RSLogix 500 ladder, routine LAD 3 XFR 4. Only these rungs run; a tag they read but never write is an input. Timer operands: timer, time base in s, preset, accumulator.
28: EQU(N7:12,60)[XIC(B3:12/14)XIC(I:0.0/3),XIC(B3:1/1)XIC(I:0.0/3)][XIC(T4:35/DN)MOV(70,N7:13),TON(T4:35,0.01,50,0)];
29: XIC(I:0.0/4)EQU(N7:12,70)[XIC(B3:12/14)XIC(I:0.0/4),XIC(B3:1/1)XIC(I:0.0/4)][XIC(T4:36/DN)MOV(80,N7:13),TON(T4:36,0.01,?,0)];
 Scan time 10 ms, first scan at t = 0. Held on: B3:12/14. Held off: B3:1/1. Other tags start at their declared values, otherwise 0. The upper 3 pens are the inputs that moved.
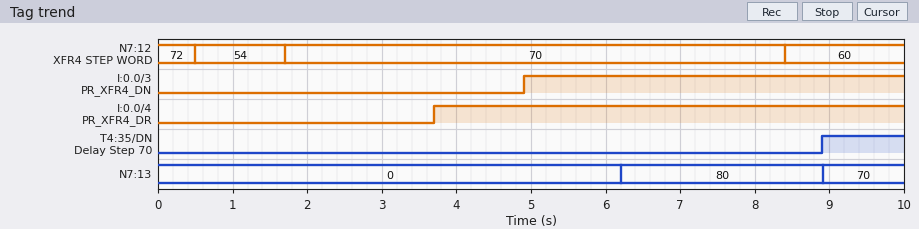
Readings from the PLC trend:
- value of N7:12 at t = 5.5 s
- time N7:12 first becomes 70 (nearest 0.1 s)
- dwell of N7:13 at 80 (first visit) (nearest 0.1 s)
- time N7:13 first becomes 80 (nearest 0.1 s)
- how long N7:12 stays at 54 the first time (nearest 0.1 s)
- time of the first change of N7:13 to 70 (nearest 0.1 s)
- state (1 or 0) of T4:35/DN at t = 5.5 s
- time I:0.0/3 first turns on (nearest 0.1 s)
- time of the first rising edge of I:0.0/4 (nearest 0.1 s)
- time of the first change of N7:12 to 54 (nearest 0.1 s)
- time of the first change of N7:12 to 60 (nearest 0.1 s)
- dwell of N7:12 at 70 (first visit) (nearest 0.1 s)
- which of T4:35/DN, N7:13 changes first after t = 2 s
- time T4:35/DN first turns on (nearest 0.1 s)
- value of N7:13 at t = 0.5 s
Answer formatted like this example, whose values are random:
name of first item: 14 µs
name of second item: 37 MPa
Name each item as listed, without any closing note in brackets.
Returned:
value of N7:12 at t = 5.5 s: 70
time N7:12 first becomes 70: 1.7 s
dwell of N7:13 at 80 (first visit): 2.7 s
time N7:13 first becomes 80: 6.2 s
how long N7:12 stays at 54 the first time: 1.2 s
time of the first change of N7:13 to 70: 8.9 s
state (1 or 0) of T4:35/DN at t = 5.5 s: 0
time I:0.0/3 first turns on: 4.9 s
time of the first rising edge of I:0.0/4: 3.7 s
time of the first change of N7:12 to 54: 0.5 s
time of the first change of N7:12 to 60: 8.4 s
dwell of N7:12 at 70 (first visit): 6.7 s
which of T4:35/DN, N7:13 changes first after t = 2 s: N7:13
time T4:35/DN first turns on: 8.9 s
value of N7:13 at t = 0.5 s: 0
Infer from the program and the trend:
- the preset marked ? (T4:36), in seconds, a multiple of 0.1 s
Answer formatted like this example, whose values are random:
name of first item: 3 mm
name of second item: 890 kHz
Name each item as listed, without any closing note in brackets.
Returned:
the preset marked ? (T4:36), in seconds, a multiple of 0.1 s: 2.5 s
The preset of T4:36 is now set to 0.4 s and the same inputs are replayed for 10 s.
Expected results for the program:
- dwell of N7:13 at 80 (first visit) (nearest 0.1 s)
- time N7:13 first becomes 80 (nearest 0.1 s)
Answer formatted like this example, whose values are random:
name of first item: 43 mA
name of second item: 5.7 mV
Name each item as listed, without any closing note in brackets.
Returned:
dwell of N7:13 at 80 (first visit): 4.8 s
time N7:13 first becomes 80: 4.1 s
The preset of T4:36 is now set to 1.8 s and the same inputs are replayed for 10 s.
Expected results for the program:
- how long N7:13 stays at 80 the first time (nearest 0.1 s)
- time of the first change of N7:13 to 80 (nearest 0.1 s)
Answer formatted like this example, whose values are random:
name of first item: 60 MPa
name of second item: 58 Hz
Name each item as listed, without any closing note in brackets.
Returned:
how long N7:13 stays at 80 the first time: 3.4 s
time of the first change of N7:13 to 80: 5.5 s
